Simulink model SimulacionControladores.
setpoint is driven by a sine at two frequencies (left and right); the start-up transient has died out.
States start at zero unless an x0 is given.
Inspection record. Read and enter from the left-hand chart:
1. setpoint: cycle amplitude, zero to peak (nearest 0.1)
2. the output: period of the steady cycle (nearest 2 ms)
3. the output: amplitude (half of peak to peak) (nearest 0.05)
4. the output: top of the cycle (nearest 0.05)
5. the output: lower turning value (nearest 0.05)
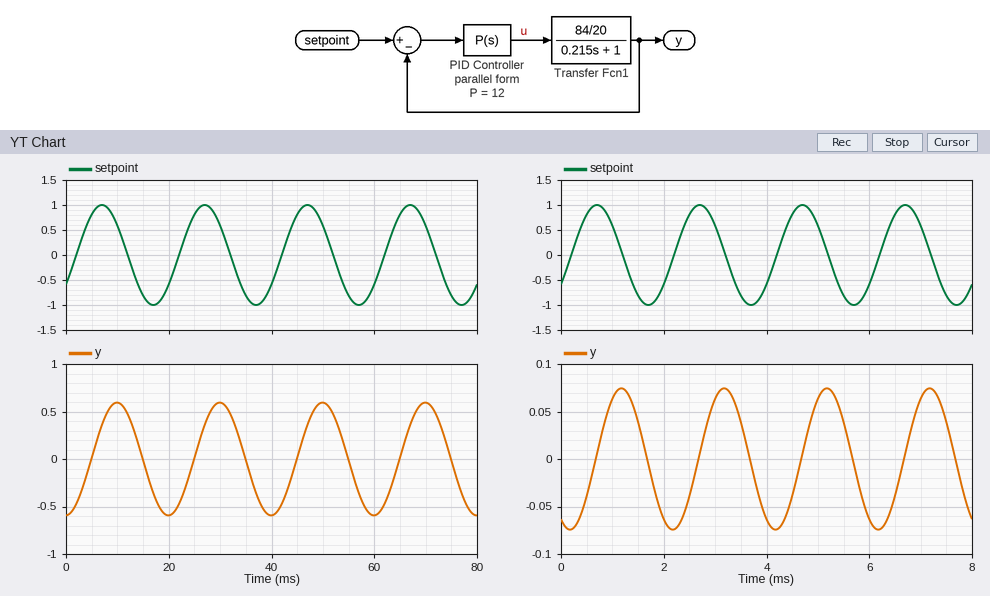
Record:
1.0
20 ms
0.60
0.60
-0.60
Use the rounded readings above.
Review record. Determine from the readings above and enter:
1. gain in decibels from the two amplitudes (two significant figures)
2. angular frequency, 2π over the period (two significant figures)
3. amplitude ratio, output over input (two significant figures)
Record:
-4.4 dB
0.31 rad/ms
0.60
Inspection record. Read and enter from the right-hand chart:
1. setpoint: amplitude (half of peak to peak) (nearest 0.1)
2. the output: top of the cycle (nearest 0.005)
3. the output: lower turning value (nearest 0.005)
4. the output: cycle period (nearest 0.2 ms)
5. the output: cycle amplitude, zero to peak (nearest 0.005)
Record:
1.0
0.075
-0.075
2.0 ms
0.075
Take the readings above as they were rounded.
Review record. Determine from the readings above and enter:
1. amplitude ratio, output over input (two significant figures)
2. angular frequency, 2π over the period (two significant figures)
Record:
0.075
3.1 rad/ms
